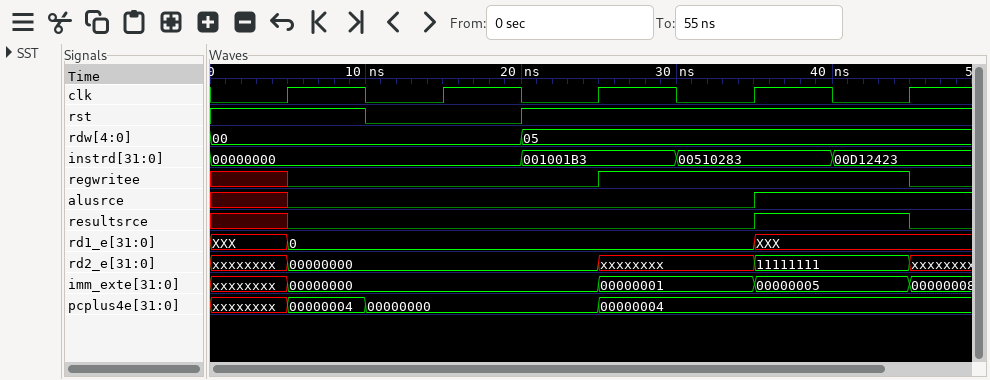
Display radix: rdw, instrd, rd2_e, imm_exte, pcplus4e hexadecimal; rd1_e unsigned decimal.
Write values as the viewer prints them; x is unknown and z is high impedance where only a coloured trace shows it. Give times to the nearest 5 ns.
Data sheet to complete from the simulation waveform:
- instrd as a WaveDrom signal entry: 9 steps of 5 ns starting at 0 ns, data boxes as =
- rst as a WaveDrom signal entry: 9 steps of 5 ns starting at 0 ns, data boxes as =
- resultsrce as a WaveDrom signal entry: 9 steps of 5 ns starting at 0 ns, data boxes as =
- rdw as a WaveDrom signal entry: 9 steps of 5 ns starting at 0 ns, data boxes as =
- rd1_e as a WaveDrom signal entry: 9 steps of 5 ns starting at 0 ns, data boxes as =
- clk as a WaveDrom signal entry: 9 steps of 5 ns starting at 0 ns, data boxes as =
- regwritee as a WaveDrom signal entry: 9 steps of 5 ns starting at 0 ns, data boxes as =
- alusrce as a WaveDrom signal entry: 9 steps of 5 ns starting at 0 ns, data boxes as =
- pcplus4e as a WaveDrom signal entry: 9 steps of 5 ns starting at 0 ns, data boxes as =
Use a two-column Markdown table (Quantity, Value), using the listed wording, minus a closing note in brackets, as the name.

| Quantity | Value |
|---|---|
| instrd as a WaveDrom signal entry: 9 steps of 5 ns starting at 0 ns, data boxes as = | {name: 'instrd', wave: '=...=.=.=', data: '00000000 001001B3 00510283 00D12423'} |
| rst as a WaveDrom signal entry: 9 steps of 5 ns starting at 0 ns, data boxes as = | {name: 'rst', wave: '1.0.1....'} |
| resultsrce as a WaveDrom signal entry: 9 steps of 5 ns starting at 0 ns, data boxes as = | {name: 'resultsrce', wave: 'x0.....1.'} |
| rdw as a WaveDrom signal entry: 9 steps of 5 ns starting at 0 ns, data boxes as = | {name: 'rdw', wave: '=...=....', data: '00 05'} |
| rd1_e as a WaveDrom signal entry: 9 steps of 5 ns starting at 0 ns, data boxes as = | {name: 'rd1_e', wave: 'x=.....x.', data: '0'} |
| clk as a WaveDrom signal entry: 9 steps of 5 ns starting at 0 ns, data boxes as = | {name: 'clk', wave: '010101010'} |
| regwritee as a WaveDrom signal entry: 9 steps of 5 ns starting at 0 ns, data boxes as = | {name: 'regwritee', wave: 'x0...1...'} |
| alusrce as a WaveDrom signal entry: 9 steps of 5 ns starting at 0 ns, data boxes as = | {name: 'alusrce', wave: 'x0.....1.'} |
| pcplus4e as a WaveDrom signal entry: 9 steps of 5 ns starting at 0 ns, data boxes as = | {name: 'pcplus4e', wave: 'x==..=...', data: '00000004 00000000 00000004'} |
